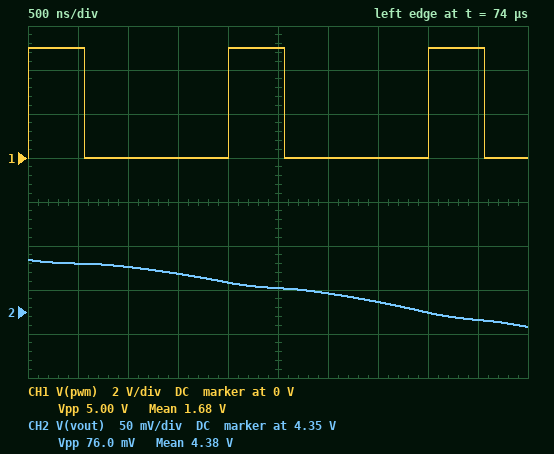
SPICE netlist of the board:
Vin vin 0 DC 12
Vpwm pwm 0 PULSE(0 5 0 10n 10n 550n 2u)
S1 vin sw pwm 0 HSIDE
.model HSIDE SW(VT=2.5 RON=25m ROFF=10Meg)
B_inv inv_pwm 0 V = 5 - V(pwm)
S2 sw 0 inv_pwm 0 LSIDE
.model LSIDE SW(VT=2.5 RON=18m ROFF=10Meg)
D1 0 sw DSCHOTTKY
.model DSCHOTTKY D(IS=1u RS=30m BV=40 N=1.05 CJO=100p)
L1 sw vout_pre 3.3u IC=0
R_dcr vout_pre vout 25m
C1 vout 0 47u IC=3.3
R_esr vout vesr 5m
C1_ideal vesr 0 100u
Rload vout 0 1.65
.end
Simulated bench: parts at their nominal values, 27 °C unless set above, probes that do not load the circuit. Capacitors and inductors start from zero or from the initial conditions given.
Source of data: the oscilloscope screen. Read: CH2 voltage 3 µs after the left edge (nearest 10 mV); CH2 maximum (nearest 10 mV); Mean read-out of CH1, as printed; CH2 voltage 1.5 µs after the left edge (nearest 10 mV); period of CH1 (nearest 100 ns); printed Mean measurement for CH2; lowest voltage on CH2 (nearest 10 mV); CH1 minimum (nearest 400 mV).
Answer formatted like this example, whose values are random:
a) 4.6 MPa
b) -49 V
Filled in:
a) 4.37 V
b) 4.41 V
c) 1.68 V
d) 4.39 V
e) 2.0 µs
f) 4.38 V
g) 4.33 V
h) 0 V
